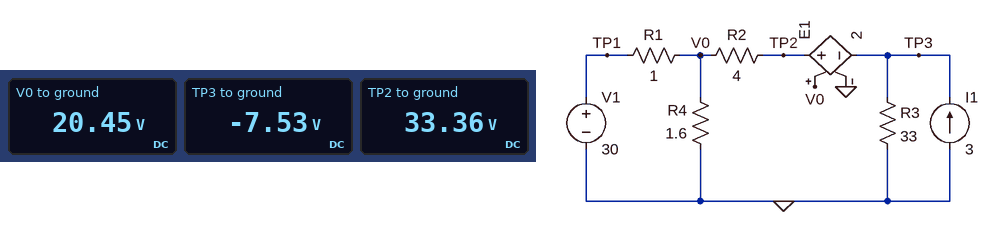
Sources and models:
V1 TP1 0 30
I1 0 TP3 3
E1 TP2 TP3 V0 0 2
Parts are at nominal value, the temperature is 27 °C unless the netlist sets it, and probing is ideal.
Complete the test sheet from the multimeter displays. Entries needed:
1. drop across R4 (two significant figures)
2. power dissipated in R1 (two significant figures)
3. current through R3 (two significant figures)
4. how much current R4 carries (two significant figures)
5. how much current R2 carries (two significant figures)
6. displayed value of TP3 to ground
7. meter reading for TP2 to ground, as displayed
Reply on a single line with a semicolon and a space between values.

20 V; 91 W; 230 mA; 13 A; 3.2 A; -7.53 V; 33.36 V
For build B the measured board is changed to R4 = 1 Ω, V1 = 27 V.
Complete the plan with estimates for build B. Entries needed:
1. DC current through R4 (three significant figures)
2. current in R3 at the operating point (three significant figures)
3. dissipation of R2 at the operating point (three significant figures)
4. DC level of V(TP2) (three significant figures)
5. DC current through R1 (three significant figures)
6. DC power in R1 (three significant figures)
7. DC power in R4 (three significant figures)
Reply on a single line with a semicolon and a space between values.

15.0 A; 82.2 mA; 38.0 W; 27.4 V; 12.0 A; 143 W; 226 W
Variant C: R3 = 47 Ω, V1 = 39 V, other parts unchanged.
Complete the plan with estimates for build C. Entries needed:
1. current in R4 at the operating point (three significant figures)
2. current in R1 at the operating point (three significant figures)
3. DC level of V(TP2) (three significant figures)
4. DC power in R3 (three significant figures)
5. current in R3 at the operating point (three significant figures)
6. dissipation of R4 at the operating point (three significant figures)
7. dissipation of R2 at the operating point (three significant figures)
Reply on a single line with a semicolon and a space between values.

16.3 A; 13.0 A; 39.1 V; 3.55 W; 275 mA; 423 W; 42.9 W
